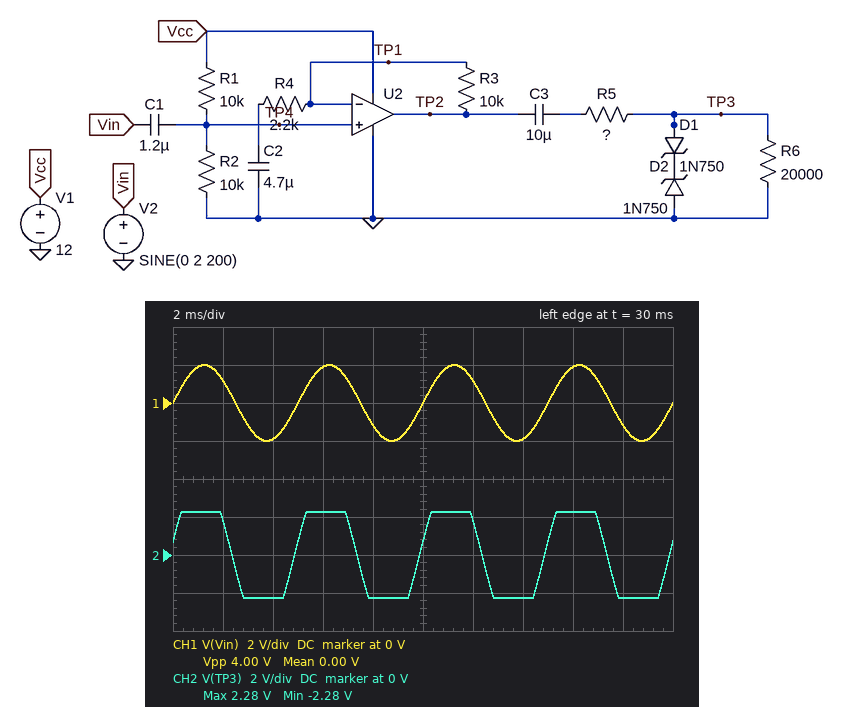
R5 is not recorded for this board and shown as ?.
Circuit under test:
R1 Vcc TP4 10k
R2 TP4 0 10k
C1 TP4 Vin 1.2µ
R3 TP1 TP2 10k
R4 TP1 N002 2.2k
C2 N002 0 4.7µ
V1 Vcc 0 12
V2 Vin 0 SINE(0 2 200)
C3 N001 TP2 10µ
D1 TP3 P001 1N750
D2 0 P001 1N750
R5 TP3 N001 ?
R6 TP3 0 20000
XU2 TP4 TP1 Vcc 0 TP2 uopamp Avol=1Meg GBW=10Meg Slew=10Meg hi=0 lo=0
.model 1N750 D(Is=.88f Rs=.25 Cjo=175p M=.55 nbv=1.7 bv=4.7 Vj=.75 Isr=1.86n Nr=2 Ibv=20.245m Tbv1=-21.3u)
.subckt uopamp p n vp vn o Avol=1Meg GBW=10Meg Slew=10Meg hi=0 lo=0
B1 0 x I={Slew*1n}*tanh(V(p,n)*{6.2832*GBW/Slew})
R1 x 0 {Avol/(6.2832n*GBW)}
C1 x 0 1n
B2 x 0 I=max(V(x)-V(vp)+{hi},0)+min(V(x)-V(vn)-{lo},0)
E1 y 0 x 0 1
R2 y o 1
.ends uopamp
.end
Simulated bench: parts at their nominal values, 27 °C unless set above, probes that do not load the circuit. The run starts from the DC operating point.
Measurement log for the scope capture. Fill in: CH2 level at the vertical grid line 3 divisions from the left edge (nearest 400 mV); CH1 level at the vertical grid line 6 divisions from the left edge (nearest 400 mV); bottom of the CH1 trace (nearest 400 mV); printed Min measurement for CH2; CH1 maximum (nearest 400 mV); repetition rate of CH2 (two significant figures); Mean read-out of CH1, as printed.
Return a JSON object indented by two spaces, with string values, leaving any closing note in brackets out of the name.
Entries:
{
  "CH2 level at the vertical grid line 3 divisions from the left edge": "2.4 V",
  "CH1 level at the vertical grid line 6 divisions from the left edge": "1.2 V",
  "bottom of the CH1 trace": "-2.0 V",
  "printed Min measurement for CH2": "-2.28 V",
  "CH1 maximum": "2.0 V",
  "repetition rate of CH2": "200 Hz",
  "Mean read-out of CH1, as printed": "0.00 V"
}
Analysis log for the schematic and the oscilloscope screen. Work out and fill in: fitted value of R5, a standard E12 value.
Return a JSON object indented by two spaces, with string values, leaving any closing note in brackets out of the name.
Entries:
{
  "fitted value of R5, a standard E12 value": "33 kΩ"
}
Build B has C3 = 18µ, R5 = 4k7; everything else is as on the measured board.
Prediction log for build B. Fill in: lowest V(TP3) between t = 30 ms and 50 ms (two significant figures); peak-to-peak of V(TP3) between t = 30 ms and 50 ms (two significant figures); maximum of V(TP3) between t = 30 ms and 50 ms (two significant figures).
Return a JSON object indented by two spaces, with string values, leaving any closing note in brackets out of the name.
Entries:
{
  "lowest V(TP3) between t = 30 ms and 50 ms": "-4.8 V",
  "peak-to-peak of V(TP3) between t = 30 ms and 50 ms": "9.7 V",
  "maximum of V(TP3) between t = 30 ms and 50 ms": "4.8 V"
}
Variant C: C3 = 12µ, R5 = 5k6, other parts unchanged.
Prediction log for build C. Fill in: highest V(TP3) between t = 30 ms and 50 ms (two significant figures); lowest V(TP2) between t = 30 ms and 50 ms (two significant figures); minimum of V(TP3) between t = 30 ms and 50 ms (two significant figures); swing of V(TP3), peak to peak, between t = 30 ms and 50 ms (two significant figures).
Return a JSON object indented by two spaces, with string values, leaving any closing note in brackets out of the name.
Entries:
{
  "highest V(TP3) between t = 30 ms and 50 ms": "4.7 V",
  "lowest V(TP2) between t = 30 ms and 50 ms": "-9.3 mV",
  "minimum of V(TP3) between t = 30 ms and 50 ms": "-4.7 V",
  "swing of V(TP3), peak to peak, between t = 30 ms and 50 ms": "9.4 V"
}
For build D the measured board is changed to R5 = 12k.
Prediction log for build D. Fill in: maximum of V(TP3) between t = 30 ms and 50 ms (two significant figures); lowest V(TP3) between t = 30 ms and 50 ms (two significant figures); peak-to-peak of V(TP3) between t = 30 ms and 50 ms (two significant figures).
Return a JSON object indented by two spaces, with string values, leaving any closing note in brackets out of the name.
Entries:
{
  "maximum of V(TP3) between t = 30 ms and 50 ms": "3.8 V",
  "lowest V(TP3) between t = 30 ms and 50 ms": "-3.8 V",
  "peak-to-peak of V(TP3) between t = 30 ms and 50 ms": "7.5 V"
}
